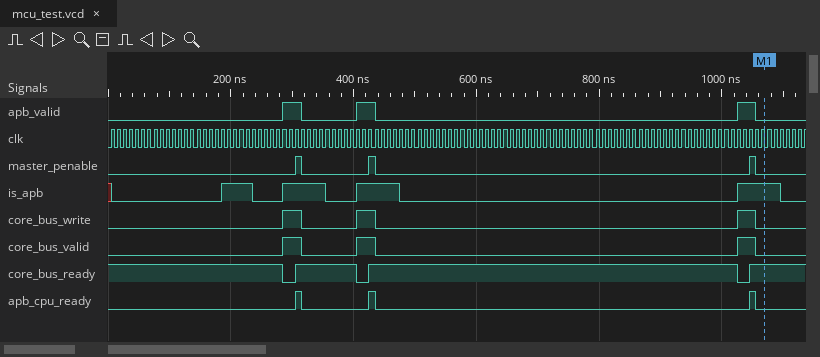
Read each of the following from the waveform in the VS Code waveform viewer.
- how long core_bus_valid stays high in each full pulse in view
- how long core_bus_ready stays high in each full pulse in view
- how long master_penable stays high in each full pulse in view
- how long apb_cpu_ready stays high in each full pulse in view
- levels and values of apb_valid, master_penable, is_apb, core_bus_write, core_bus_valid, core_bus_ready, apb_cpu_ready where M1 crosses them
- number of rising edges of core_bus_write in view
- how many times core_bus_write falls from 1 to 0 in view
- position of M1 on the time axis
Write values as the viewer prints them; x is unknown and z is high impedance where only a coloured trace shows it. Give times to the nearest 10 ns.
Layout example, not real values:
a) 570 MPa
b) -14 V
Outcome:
a) 30 ns, 30 ns, 30 ns
b) 100 ns, 600 ns
c) 10 ns, 10 ns, 10 ns
d) 10 ns, 10 ns, 10 ns
e) apb_valid=0, master_penable=0, is_apb=1, core_bus_write=0, core_bus_valid=0, core_bus_ready=1, apb_cpu_ready=0
f) 3
g) 3
h) 1070 ns
